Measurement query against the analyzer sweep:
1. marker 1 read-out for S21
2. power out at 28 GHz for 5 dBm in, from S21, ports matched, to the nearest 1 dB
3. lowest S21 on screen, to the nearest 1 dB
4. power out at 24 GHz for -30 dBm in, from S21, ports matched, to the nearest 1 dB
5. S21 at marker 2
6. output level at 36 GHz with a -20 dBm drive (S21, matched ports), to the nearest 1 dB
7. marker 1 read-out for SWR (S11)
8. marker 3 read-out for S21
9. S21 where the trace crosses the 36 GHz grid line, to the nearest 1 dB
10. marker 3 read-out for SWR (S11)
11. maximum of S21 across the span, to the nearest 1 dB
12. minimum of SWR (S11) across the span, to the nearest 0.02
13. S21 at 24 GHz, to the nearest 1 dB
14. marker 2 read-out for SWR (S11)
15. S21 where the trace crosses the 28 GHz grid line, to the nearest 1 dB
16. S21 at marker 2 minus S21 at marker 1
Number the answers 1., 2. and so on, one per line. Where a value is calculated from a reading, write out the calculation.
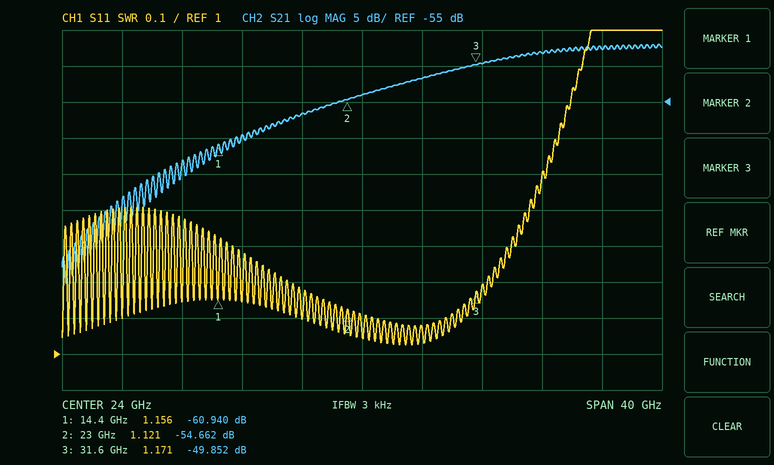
1. -60.940 dB
2. 5 dBm + (-52 dB) = -47 dBm
3. -80 dB
4. -30 dBm + (-54 dB) = -84 dBm
5. -54.662 dB
6. -20 dBm + (-48 dB) = -68 dBm
7. 1.156
8. -49.852 dB
9. -48 dB
10. 1.171
11. -47 dB
12. 1.02
13. -54 dB
14. 1.121
15. -52 dB
16. -54.662 − (-60.94) = 6.278 dB
